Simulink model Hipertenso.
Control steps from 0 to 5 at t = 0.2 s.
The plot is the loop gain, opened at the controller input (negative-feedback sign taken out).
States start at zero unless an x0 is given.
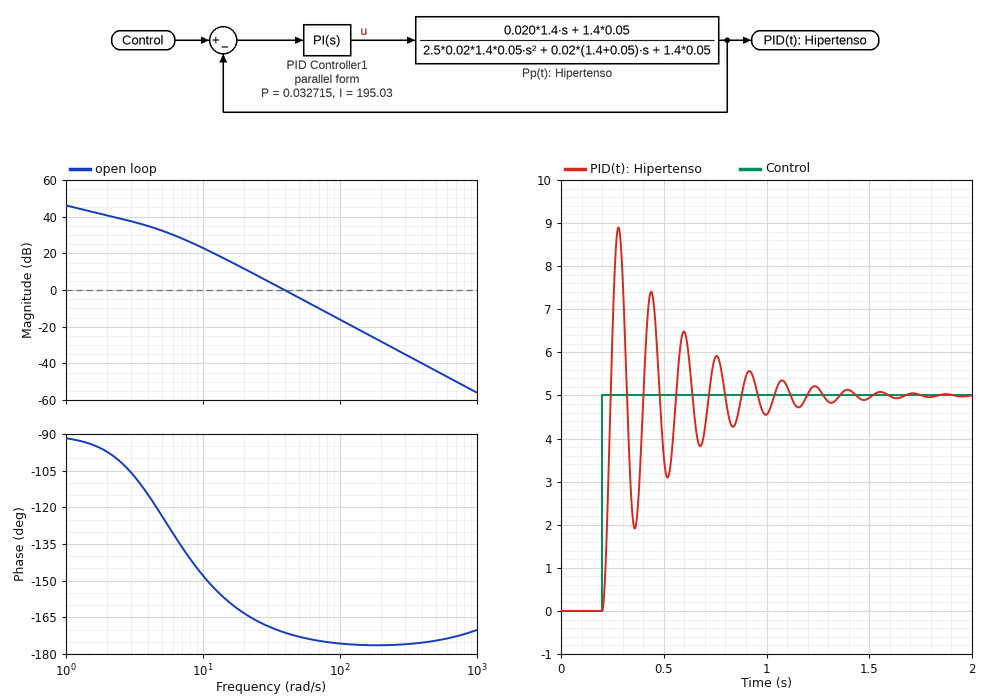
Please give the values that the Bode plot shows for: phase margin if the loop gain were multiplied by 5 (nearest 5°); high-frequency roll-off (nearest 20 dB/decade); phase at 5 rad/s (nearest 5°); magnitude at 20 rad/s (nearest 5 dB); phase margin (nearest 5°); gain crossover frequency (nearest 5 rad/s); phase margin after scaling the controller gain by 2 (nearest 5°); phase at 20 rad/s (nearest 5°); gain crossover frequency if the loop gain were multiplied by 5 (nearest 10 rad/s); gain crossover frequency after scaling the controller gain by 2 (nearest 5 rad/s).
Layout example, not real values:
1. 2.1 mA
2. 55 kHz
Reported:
1. 5°
2. -40 dB/decade
3. -125°
4. 10 dB
5. 10°
6. 40 rad/s
7. 5°
8. -165°
9. 90 rad/s
10. 55 rad/s
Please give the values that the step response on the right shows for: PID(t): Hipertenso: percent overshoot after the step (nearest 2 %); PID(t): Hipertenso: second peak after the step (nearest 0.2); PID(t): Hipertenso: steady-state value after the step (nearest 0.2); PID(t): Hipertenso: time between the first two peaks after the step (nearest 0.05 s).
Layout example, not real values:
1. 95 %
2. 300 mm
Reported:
1. 78 %
2. 7.4
3. 5.0
4. 0.15 s
